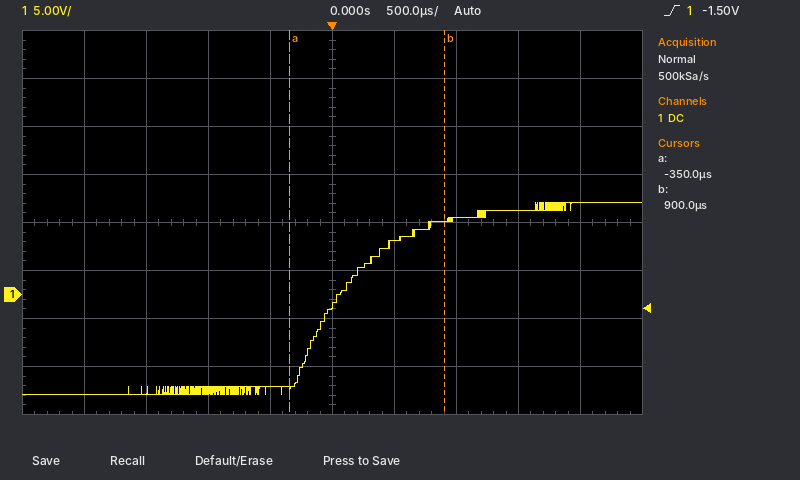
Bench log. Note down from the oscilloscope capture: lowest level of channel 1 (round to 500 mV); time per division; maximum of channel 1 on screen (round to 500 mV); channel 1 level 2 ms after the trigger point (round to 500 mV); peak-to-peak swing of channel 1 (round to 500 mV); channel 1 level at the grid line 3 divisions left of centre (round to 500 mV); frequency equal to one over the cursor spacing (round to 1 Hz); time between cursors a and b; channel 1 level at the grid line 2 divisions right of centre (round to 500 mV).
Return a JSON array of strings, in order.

["-10.5 V", "500 µs", "9.5 V", "9.5 V", "20.0 V", "-10.0 V", "800 Hz", "1.25 ms", "8.0 V"]
